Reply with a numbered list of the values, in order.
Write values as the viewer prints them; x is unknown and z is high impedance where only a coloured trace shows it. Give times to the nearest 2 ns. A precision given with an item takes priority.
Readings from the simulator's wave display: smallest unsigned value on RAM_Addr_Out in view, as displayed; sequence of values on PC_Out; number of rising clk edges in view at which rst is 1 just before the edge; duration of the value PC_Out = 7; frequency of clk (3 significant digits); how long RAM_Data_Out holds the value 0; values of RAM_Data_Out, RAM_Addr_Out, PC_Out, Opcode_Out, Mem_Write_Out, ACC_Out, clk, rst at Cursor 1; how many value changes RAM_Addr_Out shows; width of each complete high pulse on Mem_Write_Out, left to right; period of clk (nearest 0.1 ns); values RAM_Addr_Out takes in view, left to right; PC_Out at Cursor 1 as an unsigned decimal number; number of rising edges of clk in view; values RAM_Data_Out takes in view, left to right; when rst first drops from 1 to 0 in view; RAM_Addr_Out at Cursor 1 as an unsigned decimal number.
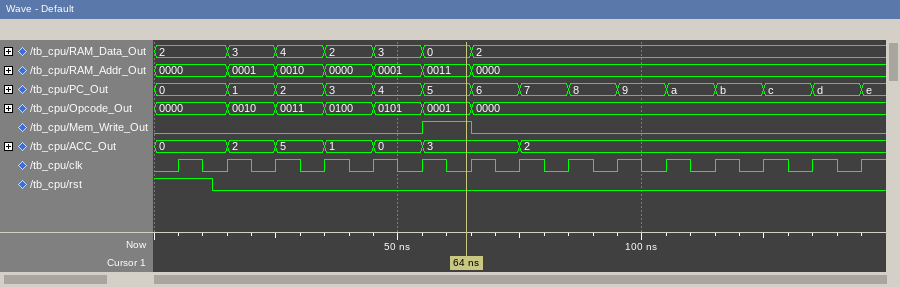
1. 0000
2. 0, 1, 2, 3, 4, 5, 6, 7, 8, 9, a, b, c, d, e
3. 1
4. 10 ns
5. 100 MHz
6. 10 ns
7. RAM_Data_Out=0, RAM_Addr_Out=0011, PC_Out=5, Opcode_Out=0001, Mem_Write_Out=1, ACC_Out=3, clk=0, rst=0
8. 6
9. 10 ns
10. 10 ns
11. 0000, 0001, 0010, 0000, 0001, 0011, 0000
12. 5
13. 15
14. 2, 3, 4, 2, 3, 0, 2
15. 12 ns
16. 3
